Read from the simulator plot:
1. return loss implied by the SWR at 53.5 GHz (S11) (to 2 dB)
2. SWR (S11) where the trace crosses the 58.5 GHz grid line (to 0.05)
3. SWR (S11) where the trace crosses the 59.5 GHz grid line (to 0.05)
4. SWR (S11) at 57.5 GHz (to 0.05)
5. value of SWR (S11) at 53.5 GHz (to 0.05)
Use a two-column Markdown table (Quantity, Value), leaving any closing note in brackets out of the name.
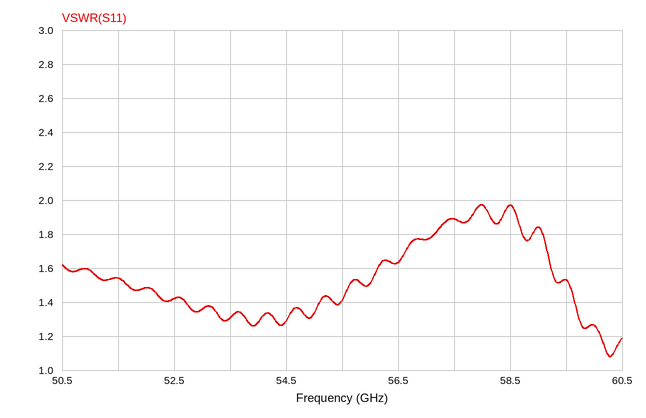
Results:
| Quantity | Value |
|---|---|
| return loss implied by the SWR at 53.5 GHz (S11) | 18 dB |
| SWR (S11) where the trace crosses the 58.5 GHz grid line | 1.95 |
| SWR (S11) where the trace crosses the 59.5 GHz grid line | 1.55 |
| SWR (S11) at 57.5 GHz | 1.90 |
| value of SWR (S11) at 53.5 GHz | 1.30 |
